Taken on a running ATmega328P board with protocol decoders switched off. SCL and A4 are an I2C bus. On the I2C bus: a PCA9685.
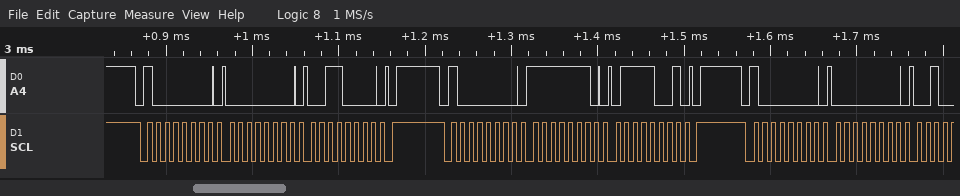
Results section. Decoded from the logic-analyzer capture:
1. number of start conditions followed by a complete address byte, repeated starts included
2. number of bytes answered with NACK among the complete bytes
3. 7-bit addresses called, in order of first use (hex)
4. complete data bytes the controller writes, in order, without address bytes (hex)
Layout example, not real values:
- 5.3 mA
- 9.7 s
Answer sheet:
- 3
- 0
- 0x40
- 00 30 FE 79 00
